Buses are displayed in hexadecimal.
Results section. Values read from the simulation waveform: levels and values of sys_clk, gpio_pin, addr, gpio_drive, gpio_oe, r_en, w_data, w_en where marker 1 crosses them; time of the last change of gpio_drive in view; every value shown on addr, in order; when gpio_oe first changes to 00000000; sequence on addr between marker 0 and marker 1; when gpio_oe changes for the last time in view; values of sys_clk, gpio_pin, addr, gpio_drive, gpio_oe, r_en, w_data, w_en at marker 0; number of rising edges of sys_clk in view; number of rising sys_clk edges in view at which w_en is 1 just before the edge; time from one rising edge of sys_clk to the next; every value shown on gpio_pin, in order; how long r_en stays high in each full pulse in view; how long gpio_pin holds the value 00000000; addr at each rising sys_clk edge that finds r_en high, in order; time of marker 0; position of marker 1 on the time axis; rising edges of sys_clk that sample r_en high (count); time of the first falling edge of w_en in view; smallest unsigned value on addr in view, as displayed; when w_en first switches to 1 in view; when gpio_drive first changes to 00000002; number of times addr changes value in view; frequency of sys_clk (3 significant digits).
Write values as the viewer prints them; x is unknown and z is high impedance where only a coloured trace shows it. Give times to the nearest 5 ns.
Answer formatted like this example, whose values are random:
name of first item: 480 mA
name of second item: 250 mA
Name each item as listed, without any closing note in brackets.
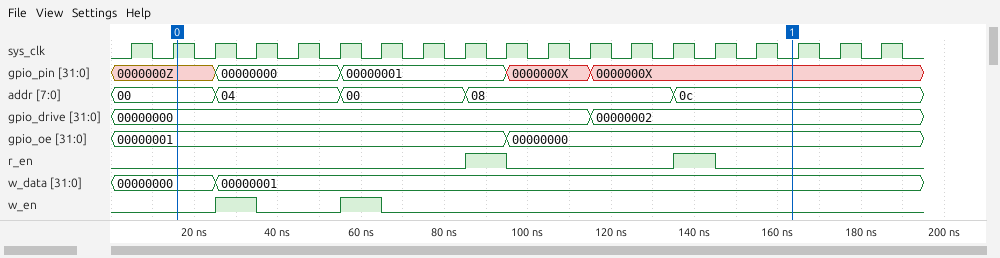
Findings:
levels and values of sys_clk, gpio_pin, addr, gpio_drive, gpio_oe, r_en, w_data, w_en where marker 1 crosses them: sys_clk=0, gpio_pin=0000000X, addr=0c, gpio_drive=00000002, gpio_oe=00000000, r_en=0, w_data=00000001, w_en=0
time of the last change of gpio_drive in view: 115 ns
every value shown on addr, in order: 00, 04, 00, 08, 0c
when gpio_oe first changes to 00000000: 95 ns
sequence on addr between marker 0 and marker 1: 00, 04, 00, 08, 0c
when gpio_oe changes for the last time in view: 95 ns
values of sys_clk, gpio_pin, addr, gpio_drive, gpio_oe, r_en, w_data, w_en at marker 0: sys_clk=1, gpio_pin=0000000Z, addr=00, gpio_drive=00000000, gpio_oe=00000001, r_en=0, w_data=00000000, w_en=0
number of rising edges of sys_clk in view: 19
number of rising sys_clk edges in view at which w_en is 1 just before the edge: 2
time from one rising edge of sys_clk to the next: 10 ns
every value shown on gpio_pin, in order: 0000000Z, 00000000, 00000001, 0000000X, 0000000X
how long r_en stays high in each full pulse in view: 10 ns, 10 ns
how long gpio_pin holds the value 00000000: 30 ns
addr at each rising sys_clk edge that finds r_en high, in order: 08, 0c
time of marker 0: 15 ns
position of marker 1 on the time axis: 165 ns
rising edges of sys_clk that sample r_en high: 2
time of the first falling edge of w_en in view: 35 ns
smallest unsigned value on addr in view, as displayed: 00
when w_en first switches to 1 in view: 25 ns
when gpio_drive first changes to 00000002: 115 ns
number of times addr changes value in view: 4
frequency of sys_clk: 100 MHz
